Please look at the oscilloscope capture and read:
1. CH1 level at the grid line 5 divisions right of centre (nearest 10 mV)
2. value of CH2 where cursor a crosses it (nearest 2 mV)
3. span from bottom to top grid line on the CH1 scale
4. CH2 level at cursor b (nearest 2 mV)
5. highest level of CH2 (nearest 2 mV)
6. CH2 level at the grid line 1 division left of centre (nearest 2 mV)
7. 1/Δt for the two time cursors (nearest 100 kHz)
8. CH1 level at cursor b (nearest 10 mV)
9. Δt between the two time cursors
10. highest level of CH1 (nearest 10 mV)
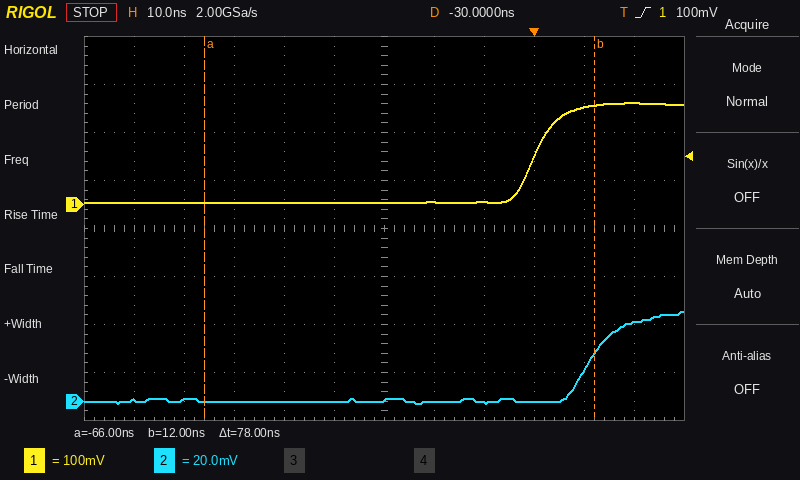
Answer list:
210 mV
0 mV
800 mV
20 mV
38 mV
0 mV
12.8 MHz
210 mV
78 ns
210 mV
